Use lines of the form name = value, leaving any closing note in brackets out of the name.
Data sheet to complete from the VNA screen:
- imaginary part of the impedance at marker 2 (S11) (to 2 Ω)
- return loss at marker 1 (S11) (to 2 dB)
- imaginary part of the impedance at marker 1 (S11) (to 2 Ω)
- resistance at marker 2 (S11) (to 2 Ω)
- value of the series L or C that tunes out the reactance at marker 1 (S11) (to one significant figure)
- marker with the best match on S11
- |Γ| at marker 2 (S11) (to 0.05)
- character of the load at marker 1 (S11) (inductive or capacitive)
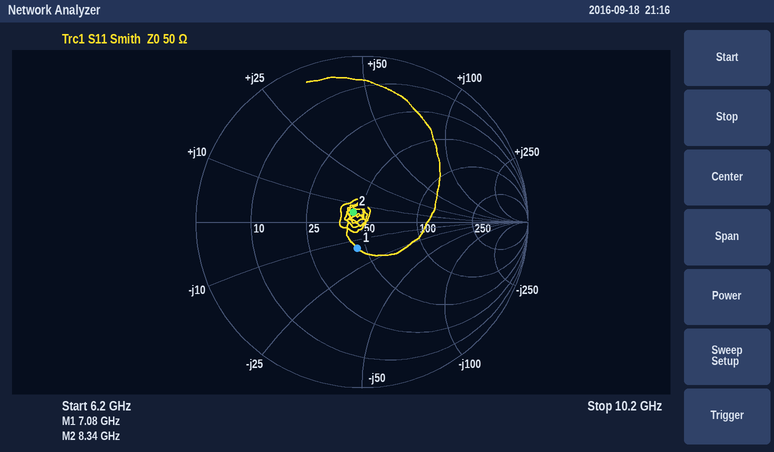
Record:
imaginary part of the impedance at marker 2 (S11) = +6 Ω
return loss at marker 1 (S11) = 16 dB
imaginary part of the impedance at marker 1 (S11) = -14 Ω
resistance at marker 2 (S11) = 44 Ω
value of the series L or C that tunes out the reactance at marker 1 (S11) = 300 pH
marker with the best match on S11 = marker 2
|Γ| at marker 2 (S11) = 0.10
character of the load at marker 1 (S11) = capacitive
